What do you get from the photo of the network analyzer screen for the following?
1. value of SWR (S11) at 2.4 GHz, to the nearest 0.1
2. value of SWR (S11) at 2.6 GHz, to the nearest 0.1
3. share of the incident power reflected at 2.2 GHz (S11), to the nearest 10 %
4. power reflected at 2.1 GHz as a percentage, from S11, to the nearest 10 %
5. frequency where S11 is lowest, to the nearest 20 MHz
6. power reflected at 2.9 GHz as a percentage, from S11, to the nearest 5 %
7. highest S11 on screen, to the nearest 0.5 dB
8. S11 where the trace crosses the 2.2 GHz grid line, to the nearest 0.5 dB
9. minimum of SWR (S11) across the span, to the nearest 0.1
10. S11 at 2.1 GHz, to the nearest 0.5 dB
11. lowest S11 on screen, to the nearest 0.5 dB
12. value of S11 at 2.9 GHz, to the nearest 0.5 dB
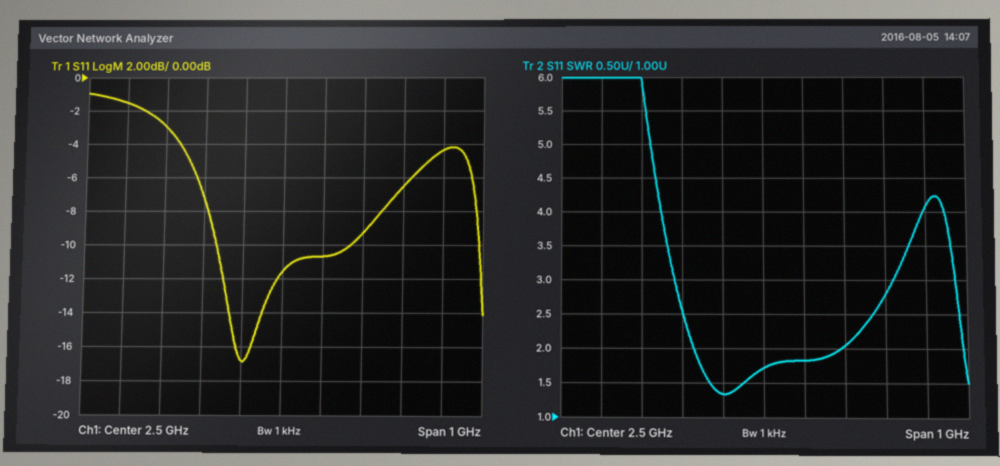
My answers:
1.3
1.8
50 %
70 %
2.40 GHz
35 %
-1.0 dB
-3.0 dB
1.3
-1.5 dB
-17.0 dB
-4.5 dB
